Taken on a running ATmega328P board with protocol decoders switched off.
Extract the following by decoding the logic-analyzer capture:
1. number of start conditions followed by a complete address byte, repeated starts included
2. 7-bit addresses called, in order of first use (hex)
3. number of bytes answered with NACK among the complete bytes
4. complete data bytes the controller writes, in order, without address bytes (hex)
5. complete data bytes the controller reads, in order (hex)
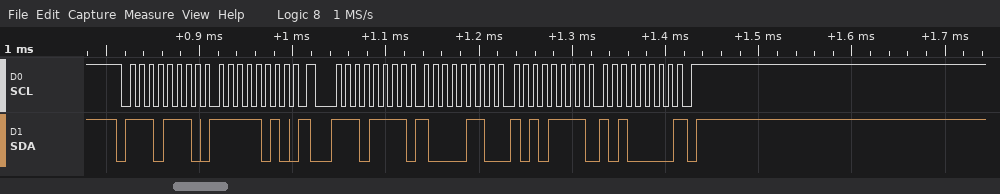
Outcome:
2
0x77
1
FA
86 AF A0
